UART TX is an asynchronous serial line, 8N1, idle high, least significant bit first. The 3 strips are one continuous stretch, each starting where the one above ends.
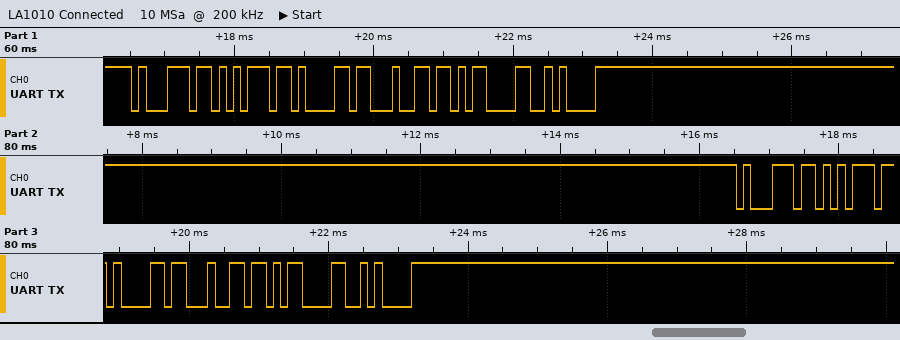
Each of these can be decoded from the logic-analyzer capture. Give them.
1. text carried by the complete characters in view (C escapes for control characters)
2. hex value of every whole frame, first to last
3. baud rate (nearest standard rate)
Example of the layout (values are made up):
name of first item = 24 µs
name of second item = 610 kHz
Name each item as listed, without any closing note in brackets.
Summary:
text carried by the complete characters in view = "quad\r\nquad\r\n"
hex value of every whole frame, first to last = 71 75 61 64 0D 0A 71 75 61 64 0D 0A
baud rate = 9600 baud
